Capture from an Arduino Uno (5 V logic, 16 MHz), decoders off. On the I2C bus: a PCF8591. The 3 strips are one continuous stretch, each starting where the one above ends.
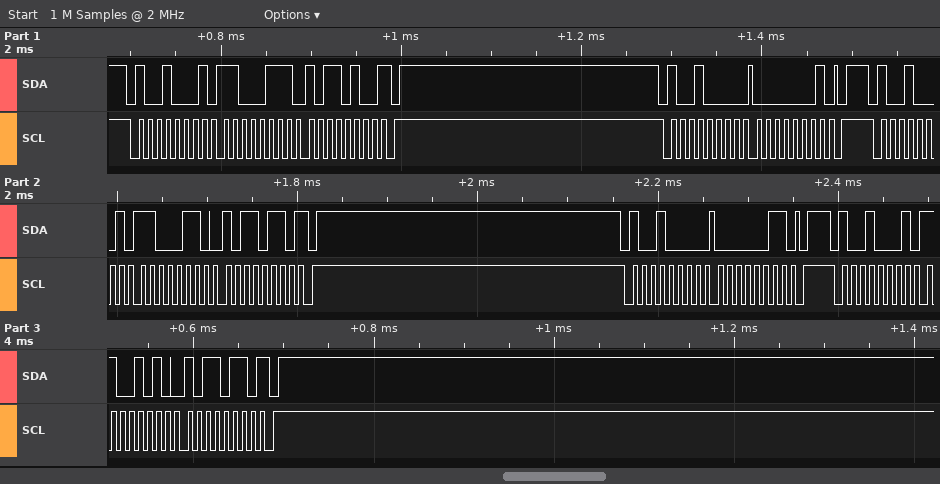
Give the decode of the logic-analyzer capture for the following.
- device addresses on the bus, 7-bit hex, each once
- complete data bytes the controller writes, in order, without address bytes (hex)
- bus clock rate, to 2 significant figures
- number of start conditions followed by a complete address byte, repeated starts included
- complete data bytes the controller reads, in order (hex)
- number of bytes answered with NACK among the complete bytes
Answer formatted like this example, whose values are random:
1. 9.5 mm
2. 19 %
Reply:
1. 0x48
2. 01 03
3. 100 kHz
4. 5
5. C7 B4 C6 B6 CA B6
6. 3
